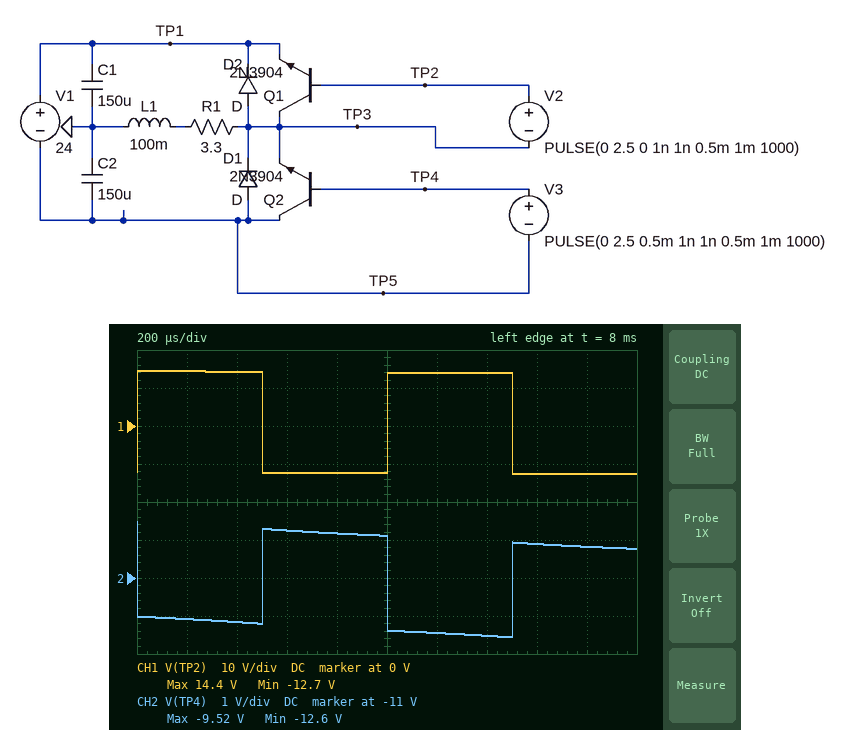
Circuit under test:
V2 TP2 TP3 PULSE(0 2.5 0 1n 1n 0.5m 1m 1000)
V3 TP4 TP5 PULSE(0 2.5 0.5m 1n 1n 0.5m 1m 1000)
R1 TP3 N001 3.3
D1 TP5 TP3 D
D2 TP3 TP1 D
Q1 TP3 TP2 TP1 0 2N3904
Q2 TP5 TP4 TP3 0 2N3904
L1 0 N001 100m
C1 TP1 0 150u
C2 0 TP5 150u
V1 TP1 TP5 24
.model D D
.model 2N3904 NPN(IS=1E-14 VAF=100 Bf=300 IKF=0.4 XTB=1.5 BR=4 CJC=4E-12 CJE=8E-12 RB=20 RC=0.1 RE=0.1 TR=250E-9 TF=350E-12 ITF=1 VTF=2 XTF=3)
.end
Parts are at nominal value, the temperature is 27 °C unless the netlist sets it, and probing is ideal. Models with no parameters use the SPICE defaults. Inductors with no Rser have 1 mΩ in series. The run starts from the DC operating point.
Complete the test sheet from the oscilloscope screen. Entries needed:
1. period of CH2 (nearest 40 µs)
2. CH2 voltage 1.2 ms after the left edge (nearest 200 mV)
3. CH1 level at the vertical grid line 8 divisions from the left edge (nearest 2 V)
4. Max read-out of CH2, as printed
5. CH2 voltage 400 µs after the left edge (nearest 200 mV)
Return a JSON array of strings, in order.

["1.00 ms", "-12.4 V", "-12 V", "-9.52 V", "-12.2 V"]
